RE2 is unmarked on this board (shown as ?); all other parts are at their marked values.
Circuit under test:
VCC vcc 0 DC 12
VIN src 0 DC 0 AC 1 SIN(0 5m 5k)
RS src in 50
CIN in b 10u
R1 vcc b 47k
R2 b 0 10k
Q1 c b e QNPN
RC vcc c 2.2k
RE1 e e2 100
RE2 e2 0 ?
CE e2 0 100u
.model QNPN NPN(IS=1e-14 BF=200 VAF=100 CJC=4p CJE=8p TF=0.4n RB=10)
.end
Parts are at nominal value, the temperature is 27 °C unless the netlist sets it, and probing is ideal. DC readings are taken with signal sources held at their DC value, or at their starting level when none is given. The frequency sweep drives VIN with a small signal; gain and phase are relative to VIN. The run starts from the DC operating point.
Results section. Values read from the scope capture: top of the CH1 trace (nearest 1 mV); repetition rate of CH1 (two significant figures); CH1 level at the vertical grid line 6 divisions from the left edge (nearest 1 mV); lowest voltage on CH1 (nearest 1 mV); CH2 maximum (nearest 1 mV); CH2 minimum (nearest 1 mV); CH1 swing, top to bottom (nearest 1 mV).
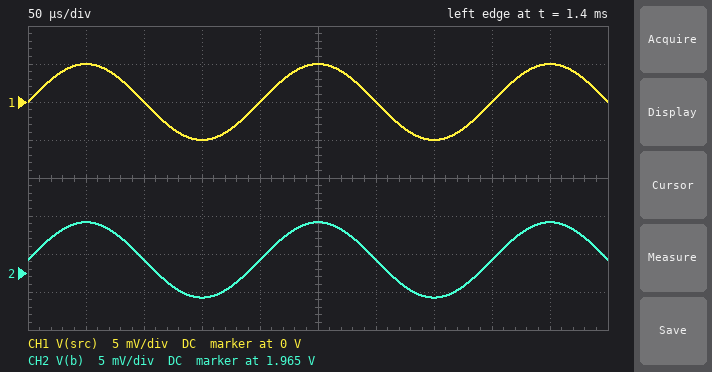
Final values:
5 mV
5.0 kHz
0 V
-5 mV
1.972 V
1.962 V
10 mV
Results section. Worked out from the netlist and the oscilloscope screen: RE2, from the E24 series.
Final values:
270 Ω
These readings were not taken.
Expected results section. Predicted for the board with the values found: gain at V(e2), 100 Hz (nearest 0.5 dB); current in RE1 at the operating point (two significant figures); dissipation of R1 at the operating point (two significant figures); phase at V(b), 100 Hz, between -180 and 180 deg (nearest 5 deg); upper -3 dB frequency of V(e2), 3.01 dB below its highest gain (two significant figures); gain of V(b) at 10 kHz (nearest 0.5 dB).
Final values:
-17.0 dB
3.5 mA
2.1 mW
0 deg
25 Hz
0 dB
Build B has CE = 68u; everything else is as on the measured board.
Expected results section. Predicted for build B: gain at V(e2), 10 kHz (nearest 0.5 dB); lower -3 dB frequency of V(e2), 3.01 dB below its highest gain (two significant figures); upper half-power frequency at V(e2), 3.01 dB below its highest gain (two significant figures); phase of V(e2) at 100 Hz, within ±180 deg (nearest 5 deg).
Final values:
-53.5 dB
1.9 Hz
35 Hz
-70 deg
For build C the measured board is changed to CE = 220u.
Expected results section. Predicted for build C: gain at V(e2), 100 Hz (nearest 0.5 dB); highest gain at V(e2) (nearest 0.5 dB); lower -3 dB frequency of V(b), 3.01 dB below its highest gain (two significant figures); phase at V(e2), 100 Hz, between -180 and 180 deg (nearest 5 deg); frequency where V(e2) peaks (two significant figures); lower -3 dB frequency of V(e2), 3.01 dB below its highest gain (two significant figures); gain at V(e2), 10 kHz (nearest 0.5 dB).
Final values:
-23.5 dB
-5.0 dB
2.3 Hz
-85 deg
4.5 Hz
1.5 Hz
-63.5 dB
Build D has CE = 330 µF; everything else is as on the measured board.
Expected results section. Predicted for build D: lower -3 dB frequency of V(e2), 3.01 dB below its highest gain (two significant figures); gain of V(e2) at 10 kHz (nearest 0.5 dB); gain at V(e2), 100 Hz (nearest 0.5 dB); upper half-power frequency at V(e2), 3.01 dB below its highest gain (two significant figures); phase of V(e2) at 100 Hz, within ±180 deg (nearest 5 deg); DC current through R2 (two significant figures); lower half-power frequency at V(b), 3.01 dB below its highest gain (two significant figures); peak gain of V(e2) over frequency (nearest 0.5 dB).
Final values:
1.3 Hz
-67.0 dB
-27.0 dB
10 Hz
-85 deg
200 µA
2.4 Hz
-6.0 dB
